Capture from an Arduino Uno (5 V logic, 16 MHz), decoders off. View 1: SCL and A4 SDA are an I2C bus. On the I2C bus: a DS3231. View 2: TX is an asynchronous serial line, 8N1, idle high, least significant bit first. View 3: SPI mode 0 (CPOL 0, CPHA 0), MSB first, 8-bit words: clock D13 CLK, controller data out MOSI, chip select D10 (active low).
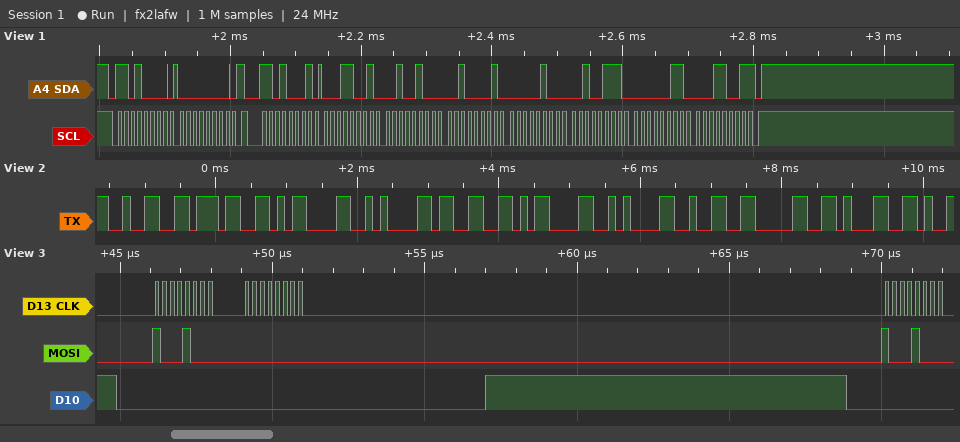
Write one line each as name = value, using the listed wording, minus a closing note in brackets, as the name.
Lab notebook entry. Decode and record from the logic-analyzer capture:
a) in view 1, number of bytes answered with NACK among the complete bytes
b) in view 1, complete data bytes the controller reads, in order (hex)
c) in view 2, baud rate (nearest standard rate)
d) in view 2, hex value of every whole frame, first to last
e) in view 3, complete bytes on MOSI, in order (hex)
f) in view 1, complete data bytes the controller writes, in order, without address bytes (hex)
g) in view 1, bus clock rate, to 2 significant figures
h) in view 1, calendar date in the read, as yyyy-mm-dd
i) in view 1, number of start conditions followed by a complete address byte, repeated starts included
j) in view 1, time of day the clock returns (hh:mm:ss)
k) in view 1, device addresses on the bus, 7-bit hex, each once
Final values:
in view 1, number of bytes answered with NACK among the complete bytes = 1
in view 1, complete data bytes the controller reads, in order = 19 24 21 04 27 03 19
in view 2, baud rate = 9600 baud
in view 2, hex value of every whole frame, first to last = 32 37 0D 0A 33 0D 0A 32 30 31
in view 3, complete bytes on MOSI, in order = 88 00 88
in view 1, complete data bytes the controller writes, in order, without address bytes = 00
in view 1, bus clock rate, to 2 significant figures = 100 kHz
in view 1, calendar date in the read, as yyyy-mm-dd = 2019-03-27
in view 1, number of start conditions followed by a complete address byte, repeated starts included = 2
in view 1, time of day the clock returns = 21:24:19
in view 1, device addresses on the bus, 7-bit hex, each once = 0x68
